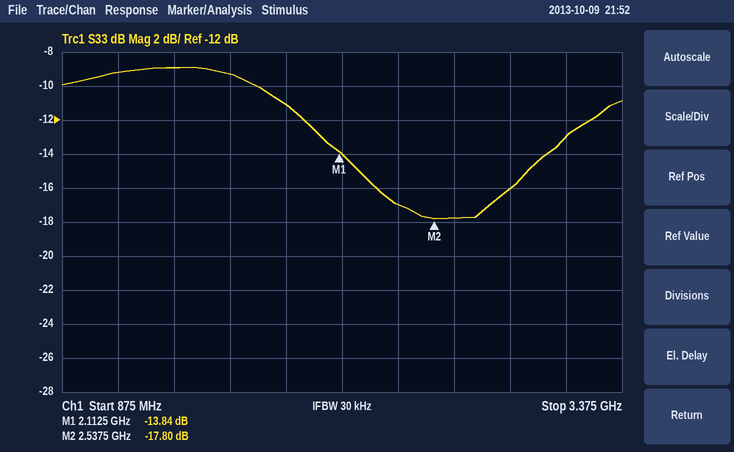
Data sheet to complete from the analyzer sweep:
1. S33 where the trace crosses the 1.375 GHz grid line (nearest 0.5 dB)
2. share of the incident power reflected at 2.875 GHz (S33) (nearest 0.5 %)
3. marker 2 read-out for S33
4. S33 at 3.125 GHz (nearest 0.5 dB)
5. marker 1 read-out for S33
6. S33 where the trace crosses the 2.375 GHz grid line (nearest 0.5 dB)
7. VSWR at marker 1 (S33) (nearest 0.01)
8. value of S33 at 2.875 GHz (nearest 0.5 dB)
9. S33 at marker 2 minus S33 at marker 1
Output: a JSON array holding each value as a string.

["-9.0 dB", "2.5 %", "-17.80 dB", "-13.0 dB", "-13.84 dB", "-17.0 dB", "1.51", "-16.0 dB", "-3.96 dB"]
